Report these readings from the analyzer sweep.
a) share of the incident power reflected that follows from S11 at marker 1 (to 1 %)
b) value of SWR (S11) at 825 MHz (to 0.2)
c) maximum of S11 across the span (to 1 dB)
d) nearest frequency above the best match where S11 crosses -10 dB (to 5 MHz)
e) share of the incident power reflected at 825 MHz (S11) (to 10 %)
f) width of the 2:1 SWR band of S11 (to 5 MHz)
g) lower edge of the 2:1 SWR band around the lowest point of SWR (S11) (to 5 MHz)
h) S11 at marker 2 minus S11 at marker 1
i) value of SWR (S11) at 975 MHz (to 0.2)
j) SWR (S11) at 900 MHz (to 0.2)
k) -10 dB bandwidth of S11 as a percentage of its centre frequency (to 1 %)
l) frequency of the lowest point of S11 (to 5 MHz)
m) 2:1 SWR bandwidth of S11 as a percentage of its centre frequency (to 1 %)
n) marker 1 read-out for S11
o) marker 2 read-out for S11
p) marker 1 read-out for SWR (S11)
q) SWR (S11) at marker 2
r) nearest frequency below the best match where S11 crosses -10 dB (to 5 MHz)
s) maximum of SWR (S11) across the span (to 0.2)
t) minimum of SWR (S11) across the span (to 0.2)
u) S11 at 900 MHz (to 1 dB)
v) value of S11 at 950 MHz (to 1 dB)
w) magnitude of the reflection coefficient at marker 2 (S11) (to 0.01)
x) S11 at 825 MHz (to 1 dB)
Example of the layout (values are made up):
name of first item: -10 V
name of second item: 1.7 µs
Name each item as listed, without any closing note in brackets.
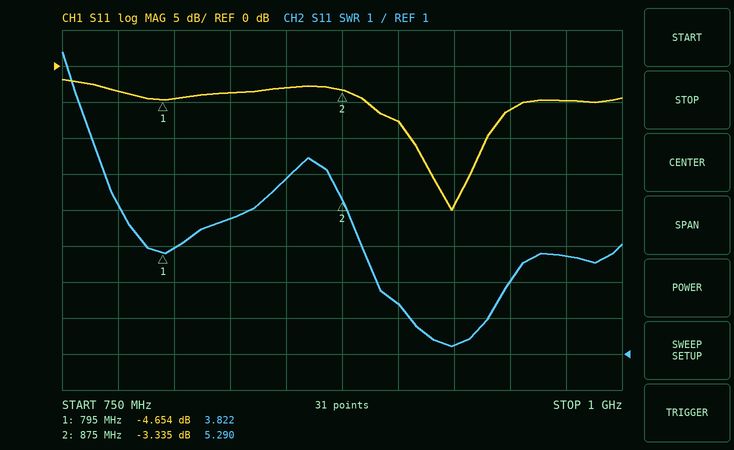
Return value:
share of the incident power reflected that follows from S11 at marker 1: 34 %
value of SWR (S11) at 825 MHz: 4.8
maximum of S11 across the span: -2 dB
nearest frequency above the best match where S11 crosses -10 dB: 940 MHz
share of the incident power reflected at 825 MHz (S11): 40 %
width of the 2:1 SWR band of S11: 35 MHz
lower edge of the 2:1 SWR band around the lowest point of SWR (S11): 905 MHz
S11 at marker 2 minus S11 at marker 1: 1.319 dB
value of SWR (S11) at 975 MHz: 3.8
SWR (S11) at 900 MHz: 2.4
-10 dB bandwidth of S11 as a percentage of its centre frequency: 4 %
frequency of the lowest point of S11: 925 MHz
2:1 SWR bandwidth of S11 as a percentage of its centre frequency: 4 %
marker 1 read-out for S11: -4.654 dB
marker 2 read-out for S11: -3.335 dB
marker 1 read-out for SWR: 3.822
SWR (S11) at marker 2: 5.290
nearest frequency below the best match where S11 crosses -10 dB: 905 MHz
maximum of SWR (S11) across the span: 9.4
minimum of SWR (S11) across the span: 1.2
S11 at 900 MHz: -8 dB
value of S11 at 950 MHz: -6 dB
magnitude of the reflection coefficient at marker 2 (S11): 0.68
S11 at 825 MHz: -4 dB
